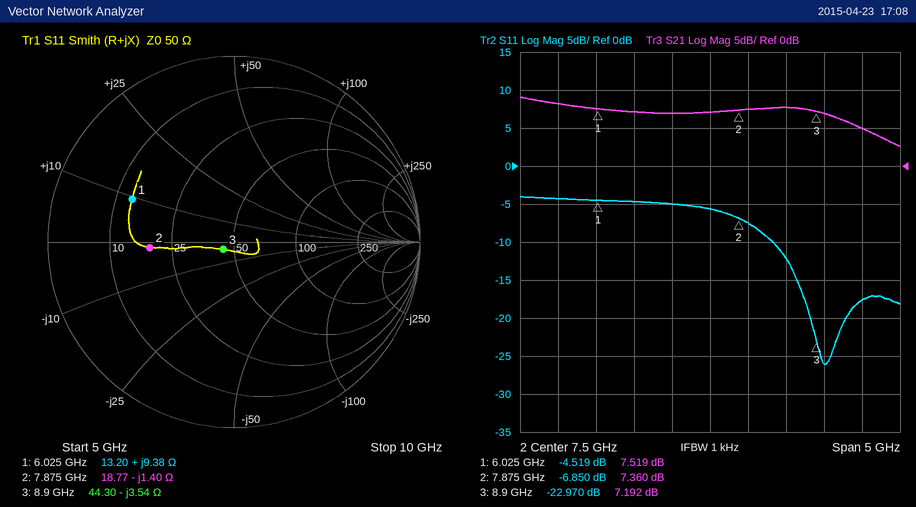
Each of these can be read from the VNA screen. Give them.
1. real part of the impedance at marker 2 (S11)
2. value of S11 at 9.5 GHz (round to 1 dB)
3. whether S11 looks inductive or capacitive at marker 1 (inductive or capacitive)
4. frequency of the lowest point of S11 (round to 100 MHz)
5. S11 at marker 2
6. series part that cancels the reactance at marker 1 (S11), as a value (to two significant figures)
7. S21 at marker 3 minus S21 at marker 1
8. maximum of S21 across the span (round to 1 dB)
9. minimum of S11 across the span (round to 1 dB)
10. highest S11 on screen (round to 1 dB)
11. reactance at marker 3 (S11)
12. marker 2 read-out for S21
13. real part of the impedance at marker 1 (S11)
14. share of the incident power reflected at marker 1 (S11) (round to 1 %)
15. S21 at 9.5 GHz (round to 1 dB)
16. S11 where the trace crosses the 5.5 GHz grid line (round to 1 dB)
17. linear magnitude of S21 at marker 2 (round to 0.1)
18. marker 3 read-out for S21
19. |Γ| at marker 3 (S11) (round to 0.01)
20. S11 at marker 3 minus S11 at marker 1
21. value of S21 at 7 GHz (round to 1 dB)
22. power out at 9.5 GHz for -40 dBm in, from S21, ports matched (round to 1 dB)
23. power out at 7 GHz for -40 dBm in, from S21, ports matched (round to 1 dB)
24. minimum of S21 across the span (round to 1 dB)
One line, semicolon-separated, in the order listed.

18.77 Ω; -18 dB; inductive; 9.0 GHz; -6.850 dB; 2.8 pF; -0.327 dB; 9 dB; -26 dB; -4 dB; -3.54 Ω; 7.360 dB; 13.20 Ω; 35 %; 5 dB; -4 dB; 2.3; 7.192 dB; 0.07; -18.451 dB; 7 dB; -35 dBm; -33 dBm; 3 dB
